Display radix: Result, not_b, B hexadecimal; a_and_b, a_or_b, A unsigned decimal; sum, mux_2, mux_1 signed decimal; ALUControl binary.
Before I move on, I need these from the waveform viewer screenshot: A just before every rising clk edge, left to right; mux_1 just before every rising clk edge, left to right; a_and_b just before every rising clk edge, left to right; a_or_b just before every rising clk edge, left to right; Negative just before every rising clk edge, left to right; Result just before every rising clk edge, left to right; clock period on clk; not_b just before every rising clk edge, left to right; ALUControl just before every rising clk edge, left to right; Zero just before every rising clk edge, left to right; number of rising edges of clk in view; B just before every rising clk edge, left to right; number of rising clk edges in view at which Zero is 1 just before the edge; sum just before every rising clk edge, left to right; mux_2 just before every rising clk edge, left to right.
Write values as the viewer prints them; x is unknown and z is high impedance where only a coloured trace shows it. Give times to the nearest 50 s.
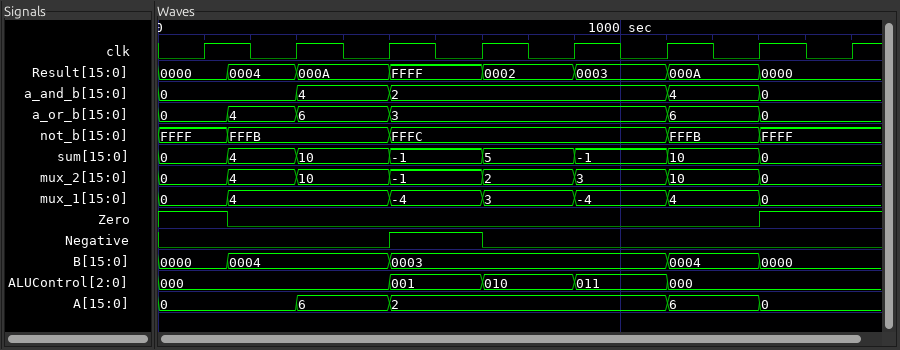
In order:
0, 0, 6, 2, 2, 2, 6, 0
0, 4, 4, -4, 3, -4, 4, 0
0, 0, 4, 2, 2, 2, 4, 0
0, 4, 6, 3, 3, 3, 6, 0
0 0 0 1 0 0 0 0
0000, 0004, 000A, FFFF, 0002, 0003, 000A, 0000
200 s
FFFF, FFFB, FFFB, FFFC, FFFC, FFFC, FFFB, FFFF
000, 000, 000, 001, 010, 011, 000, 000
1 0 0 0 0 0 0 1
8
0000, 0004, 0004, 0003, 0003, 0003, 0004, 0000
2
0, 4, 10, -1, 5, -1, 10, 0
0, 4, 10, -1, 2, 3, 10, 0
